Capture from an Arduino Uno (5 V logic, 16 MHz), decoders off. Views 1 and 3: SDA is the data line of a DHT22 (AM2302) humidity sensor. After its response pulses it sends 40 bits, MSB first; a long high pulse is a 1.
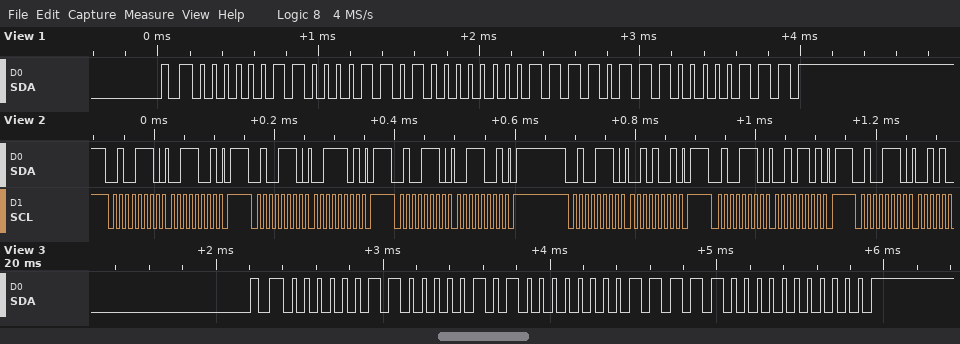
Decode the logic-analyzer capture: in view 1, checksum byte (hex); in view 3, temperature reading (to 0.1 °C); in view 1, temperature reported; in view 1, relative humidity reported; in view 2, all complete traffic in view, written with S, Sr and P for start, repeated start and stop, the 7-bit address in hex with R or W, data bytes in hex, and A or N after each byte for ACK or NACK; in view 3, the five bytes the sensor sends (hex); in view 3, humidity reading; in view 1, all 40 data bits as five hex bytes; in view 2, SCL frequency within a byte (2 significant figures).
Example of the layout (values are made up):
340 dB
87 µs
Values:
0x07
24.8 °C
24.7 °C
78.1 %
S 27W A 39 A P S 27W A 3D A P S 27W A 39 A P S 27W A 29 A P S 27W A 2D A P S 27W A
03 05 00 F8 00
77.3 %
03 0D 00 F7 07
100 kHz
